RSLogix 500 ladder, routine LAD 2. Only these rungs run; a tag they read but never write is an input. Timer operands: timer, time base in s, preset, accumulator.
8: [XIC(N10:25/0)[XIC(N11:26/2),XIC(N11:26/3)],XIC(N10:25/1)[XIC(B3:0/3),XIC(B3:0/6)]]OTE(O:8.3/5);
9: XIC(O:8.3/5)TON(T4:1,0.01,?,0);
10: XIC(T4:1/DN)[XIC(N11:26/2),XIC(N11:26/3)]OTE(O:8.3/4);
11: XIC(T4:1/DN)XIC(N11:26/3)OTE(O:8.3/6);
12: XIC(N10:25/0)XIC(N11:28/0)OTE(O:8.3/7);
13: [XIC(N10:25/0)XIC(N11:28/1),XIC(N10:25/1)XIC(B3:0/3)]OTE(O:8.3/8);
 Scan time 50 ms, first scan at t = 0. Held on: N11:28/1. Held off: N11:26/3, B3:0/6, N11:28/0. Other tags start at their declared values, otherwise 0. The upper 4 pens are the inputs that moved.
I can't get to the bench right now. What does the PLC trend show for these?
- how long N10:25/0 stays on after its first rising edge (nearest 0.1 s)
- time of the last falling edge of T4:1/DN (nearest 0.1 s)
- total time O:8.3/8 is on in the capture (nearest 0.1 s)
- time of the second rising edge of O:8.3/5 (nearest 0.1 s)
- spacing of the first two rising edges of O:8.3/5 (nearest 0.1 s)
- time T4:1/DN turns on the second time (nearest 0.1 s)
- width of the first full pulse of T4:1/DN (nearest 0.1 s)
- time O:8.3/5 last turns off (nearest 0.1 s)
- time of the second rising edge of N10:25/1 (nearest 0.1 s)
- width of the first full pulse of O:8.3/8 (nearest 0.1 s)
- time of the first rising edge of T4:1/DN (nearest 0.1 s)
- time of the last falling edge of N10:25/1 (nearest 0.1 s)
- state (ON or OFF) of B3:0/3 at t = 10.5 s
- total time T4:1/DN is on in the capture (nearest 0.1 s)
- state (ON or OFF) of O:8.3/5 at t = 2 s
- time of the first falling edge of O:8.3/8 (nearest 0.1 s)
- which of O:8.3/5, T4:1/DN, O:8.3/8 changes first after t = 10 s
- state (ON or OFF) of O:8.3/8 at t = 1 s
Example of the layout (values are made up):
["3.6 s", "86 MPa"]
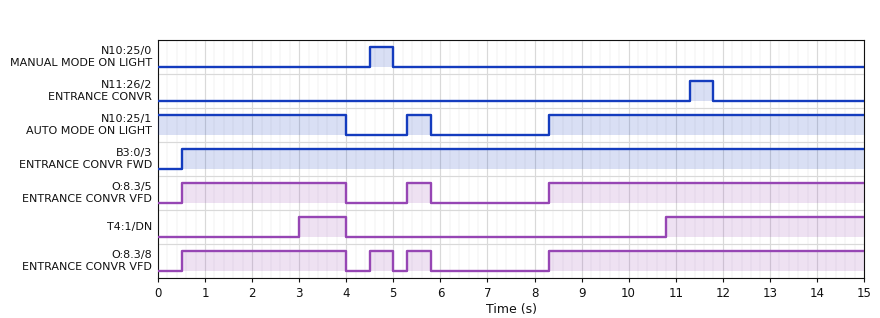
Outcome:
["0.5 s", "4.0 s", "11.2 s", "5.3 s", "4.8 s", "10.8 s", "1.0 s", "5.8 s", "8.3 s", "3.5 s", "3.0 s", "5.8 s", "ON", "5.2 s", "ON", "4.0 s", "T4:1/DN", "ON"]
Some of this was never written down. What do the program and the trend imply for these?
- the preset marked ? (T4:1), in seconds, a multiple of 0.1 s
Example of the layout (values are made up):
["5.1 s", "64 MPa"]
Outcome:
["2.5 s"]
